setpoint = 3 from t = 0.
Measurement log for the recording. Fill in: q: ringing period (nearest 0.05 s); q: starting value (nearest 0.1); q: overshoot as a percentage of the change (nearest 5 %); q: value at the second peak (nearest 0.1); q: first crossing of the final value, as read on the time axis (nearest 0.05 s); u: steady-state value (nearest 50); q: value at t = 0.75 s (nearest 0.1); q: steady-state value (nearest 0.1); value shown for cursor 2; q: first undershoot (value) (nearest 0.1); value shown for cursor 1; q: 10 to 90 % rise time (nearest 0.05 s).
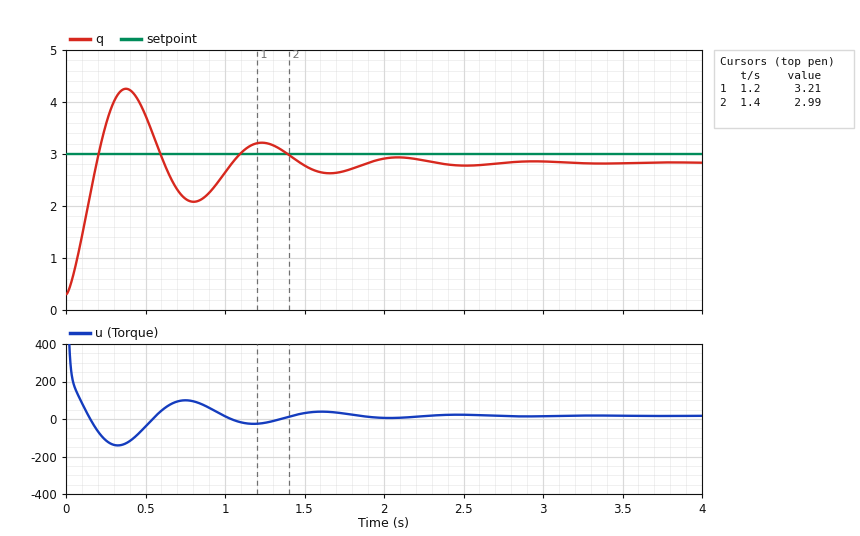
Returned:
0.85 s
0.3
55 %
3.2
0.20 s
0
2.1
2.8
2.99
2.1
3.21
0.15 s
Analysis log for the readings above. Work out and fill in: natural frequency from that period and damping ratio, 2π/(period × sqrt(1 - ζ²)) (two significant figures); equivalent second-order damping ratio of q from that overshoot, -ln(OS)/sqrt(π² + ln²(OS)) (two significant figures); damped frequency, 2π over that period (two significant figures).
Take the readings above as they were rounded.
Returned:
7.5 rad/s
0.19
7.4 rad/s
